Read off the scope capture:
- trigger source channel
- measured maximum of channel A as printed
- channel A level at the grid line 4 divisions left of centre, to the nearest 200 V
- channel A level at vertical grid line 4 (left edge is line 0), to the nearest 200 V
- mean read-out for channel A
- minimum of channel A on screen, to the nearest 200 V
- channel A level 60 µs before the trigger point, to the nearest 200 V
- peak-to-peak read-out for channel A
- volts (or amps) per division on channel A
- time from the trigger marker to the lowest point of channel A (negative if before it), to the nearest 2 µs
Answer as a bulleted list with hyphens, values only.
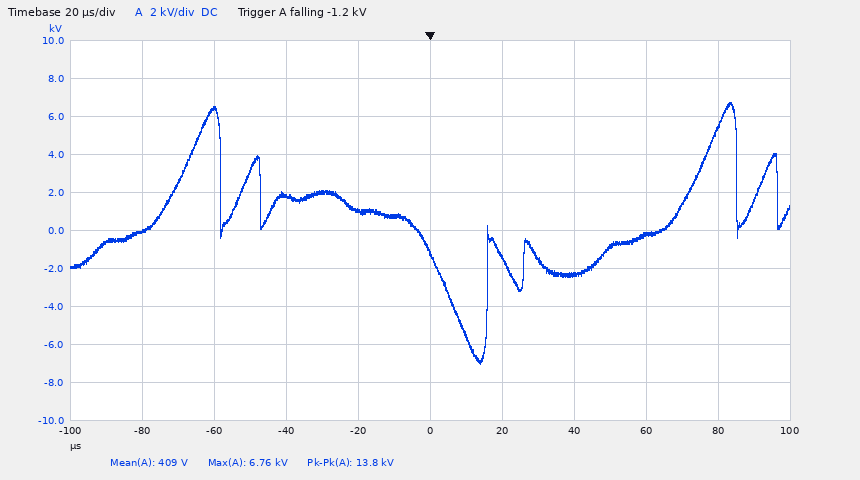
- channel A
- 6.76 kV
- 0.0 kV
- 1.0 kV
- 409 V
- -7.0 kV
- 6.4 kV
- 13.8 kV
- 2 kV
- +14 µs
